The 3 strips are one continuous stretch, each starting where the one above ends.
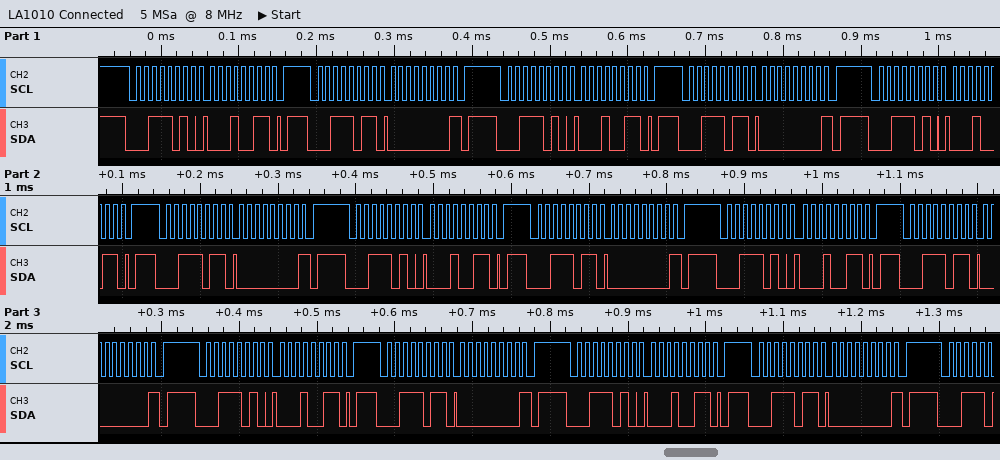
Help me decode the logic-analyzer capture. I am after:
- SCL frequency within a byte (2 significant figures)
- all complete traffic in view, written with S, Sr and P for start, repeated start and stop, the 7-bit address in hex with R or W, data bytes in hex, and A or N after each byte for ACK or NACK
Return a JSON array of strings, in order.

["100 kHz", "S 1DW A 13 A P S 1DR A 00 N P S 1DW A 13 A P S 1DR A 00 N P S 1DW A 13 A P S 1DR A 00 N P S 1DW A 13 A P S 1DR A 00 N P S 1DW A 13 A P S 1DR A 00 N P S 1DW A 13 A P S 1DR A 00 N P S 1DW A 13 A P S 1DR A 00 N P"]
